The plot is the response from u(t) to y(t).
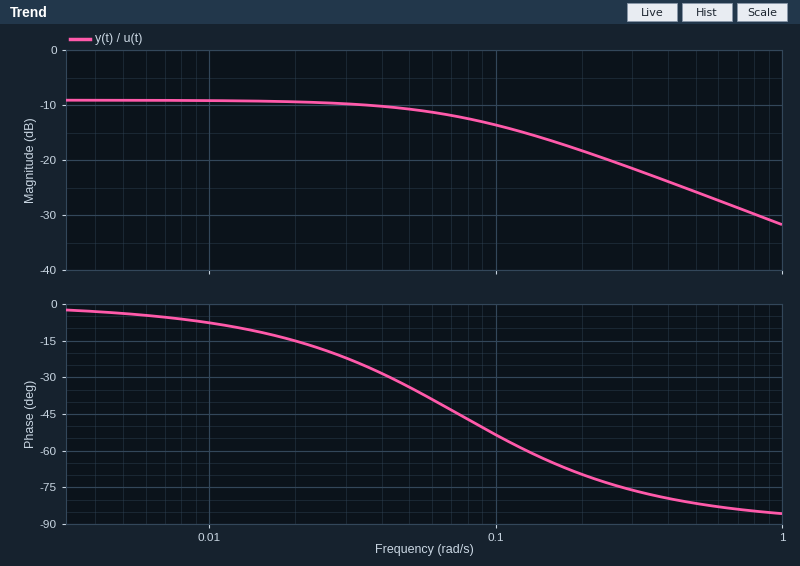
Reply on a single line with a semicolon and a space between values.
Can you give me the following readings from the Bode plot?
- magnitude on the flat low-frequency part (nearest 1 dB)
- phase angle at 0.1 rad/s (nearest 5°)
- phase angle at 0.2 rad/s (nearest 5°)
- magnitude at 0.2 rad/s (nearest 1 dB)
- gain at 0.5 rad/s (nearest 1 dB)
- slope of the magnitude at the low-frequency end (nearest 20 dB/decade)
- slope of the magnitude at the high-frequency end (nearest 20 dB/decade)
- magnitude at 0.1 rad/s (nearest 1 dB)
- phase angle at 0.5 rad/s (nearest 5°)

-9 dB; -55°; -70°; -18 dB; -26 dB; 0 dB/decade; -20 dB/decade; -14 dB; -80°
